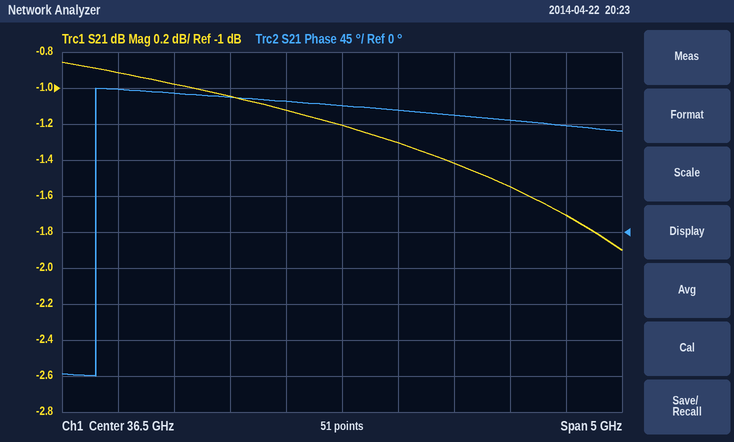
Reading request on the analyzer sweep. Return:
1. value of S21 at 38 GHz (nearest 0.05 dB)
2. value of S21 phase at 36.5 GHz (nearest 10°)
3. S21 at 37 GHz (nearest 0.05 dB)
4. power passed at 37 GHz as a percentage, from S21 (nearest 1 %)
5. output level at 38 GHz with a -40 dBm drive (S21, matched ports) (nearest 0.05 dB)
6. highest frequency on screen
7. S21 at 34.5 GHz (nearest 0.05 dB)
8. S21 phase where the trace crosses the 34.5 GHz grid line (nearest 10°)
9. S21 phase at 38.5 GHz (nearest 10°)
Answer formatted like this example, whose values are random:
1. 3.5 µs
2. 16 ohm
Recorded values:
1. -1.55 dB
2. 160°
3. -1.30 dB
4. 74 %
5. -41.55 dBm
6. 39 GHz
7. -0.90 dB
8. 180°
9. 130°
